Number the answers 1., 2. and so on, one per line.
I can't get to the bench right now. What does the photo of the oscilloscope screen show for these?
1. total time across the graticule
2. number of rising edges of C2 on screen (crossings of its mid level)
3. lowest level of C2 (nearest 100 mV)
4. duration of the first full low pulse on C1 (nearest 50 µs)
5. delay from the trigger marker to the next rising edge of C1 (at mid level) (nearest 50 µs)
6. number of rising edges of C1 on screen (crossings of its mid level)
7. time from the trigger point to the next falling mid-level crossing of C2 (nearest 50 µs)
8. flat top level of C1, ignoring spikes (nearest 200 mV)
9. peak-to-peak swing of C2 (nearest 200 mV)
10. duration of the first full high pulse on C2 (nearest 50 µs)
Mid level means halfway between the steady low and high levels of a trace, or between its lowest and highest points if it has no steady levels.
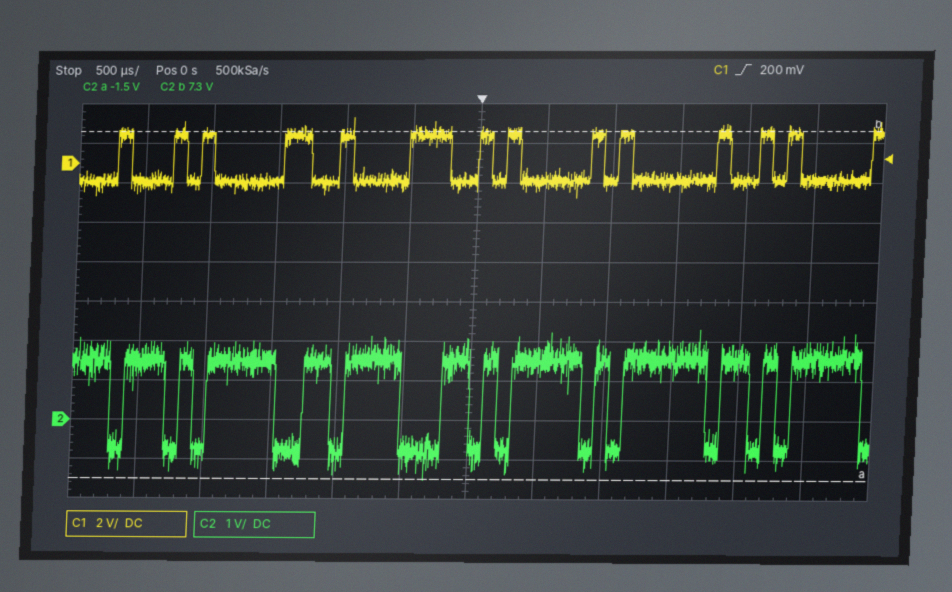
1. 6 ms
2. 13
3. -1.5 V
4. 300 µs
5. 200 µs
6. 14
7. 200 µs
8. 1.4 V
9. 3.8 V
10. 300 µs
